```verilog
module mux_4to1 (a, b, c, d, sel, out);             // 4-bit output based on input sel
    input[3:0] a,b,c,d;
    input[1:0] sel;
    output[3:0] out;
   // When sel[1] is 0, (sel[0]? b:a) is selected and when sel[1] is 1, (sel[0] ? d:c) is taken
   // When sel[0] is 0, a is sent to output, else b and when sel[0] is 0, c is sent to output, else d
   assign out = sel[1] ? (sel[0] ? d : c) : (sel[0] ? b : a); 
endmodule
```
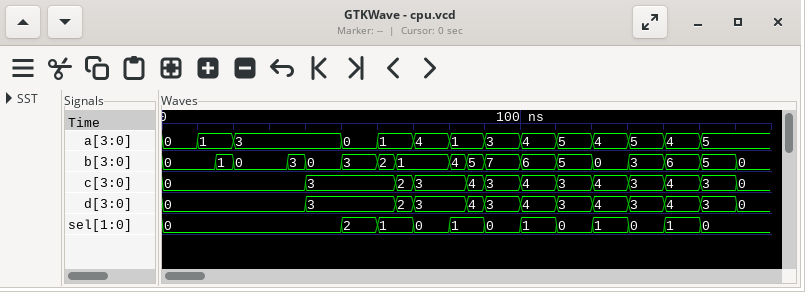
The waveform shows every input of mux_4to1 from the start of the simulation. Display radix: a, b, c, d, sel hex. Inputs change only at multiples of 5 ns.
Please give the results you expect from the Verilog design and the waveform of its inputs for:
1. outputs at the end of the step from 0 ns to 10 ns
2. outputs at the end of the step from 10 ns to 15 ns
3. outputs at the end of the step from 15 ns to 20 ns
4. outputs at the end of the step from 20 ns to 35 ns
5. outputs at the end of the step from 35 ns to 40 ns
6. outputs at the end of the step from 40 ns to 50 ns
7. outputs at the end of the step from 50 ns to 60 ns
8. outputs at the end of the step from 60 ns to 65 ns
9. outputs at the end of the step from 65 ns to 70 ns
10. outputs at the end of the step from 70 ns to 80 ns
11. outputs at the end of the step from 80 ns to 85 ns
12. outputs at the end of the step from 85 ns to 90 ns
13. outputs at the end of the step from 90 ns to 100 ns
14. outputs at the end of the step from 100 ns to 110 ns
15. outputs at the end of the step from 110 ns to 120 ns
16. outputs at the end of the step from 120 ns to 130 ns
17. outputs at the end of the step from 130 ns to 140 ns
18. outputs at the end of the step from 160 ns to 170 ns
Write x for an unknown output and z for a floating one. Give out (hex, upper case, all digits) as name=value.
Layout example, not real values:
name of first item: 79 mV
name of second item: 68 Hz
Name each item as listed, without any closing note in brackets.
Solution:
outputs at the end of the step from 0 ns to 10 ns: out=0
outputs at the end of the step from 10 ns to 15 ns: out=1
outputs at the end of the step from 15 ns to 20 ns: out=1
outputs at the end of the step from 20 ns to 35 ns: out=3
outputs at the end of the step from 35 ns to 40 ns: out=3
outputs at the end of the step from 40 ns to 50 ns: out=3
outputs at the end of the step from 50 ns to 60 ns: out=3
outputs at the end of the step from 60 ns to 65 ns: out=2
outputs at the end of the step from 65 ns to 70 ns: out=1
outputs at the end of the step from 70 ns to 80 ns: out=4
outputs at the end of the step from 80 ns to 85 ns: out=4
outputs at the end of the step from 85 ns to 90 ns: out=5
outputs at the end of the step from 90 ns to 100 ns: out=3
outputs at the end of the step from 100 ns to 110 ns: out=6
outputs at the end of the step from 110 ns to 120 ns: out=5
outputs at the end of the step from 120 ns to 130 ns: out=0
outputs at the end of the step from 130 ns to 140 ns: out=5
outputs at the end of the step from 160 ns to 170 ns: out=5
